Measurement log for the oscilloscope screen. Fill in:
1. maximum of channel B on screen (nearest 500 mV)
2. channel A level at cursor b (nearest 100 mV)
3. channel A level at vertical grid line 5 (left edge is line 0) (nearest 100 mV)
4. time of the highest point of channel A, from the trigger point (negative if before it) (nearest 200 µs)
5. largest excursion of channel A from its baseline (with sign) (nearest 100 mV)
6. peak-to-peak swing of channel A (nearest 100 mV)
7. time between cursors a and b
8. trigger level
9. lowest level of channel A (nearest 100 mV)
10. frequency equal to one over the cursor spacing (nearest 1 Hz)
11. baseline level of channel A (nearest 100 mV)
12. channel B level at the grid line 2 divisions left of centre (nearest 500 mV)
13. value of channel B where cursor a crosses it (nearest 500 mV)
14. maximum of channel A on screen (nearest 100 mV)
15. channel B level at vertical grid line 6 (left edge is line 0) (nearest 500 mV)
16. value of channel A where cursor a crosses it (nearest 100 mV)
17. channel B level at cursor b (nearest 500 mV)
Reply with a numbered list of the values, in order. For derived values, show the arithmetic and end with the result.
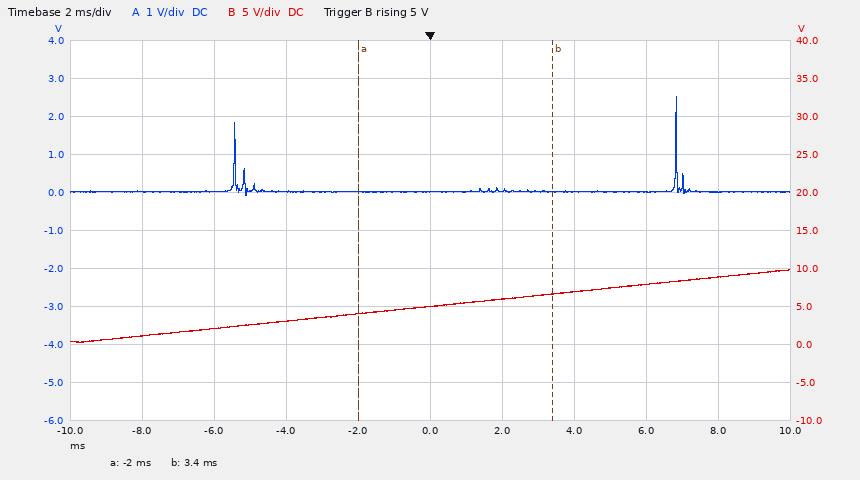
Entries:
1. 10.0 V
2. 0.0 V
3. 0.0 V
4. +6.8 ms
5. 2.5 V − (0.0 V) = +2.5 V
6. 2.5 V − (-100 mV) = 2.6 V
7. 3.4 ms − (-2 ms) = 5.4 ms
8. 5 V
9. -100 mV
10. 1 / 5.4 ms ≈ 185 Hz
11. 0.0 V
12. 3.0 V
13. 4.0 V
14. 2.5 V
15. 6.0 V
16. 0.0 V
17. 6.5 V
